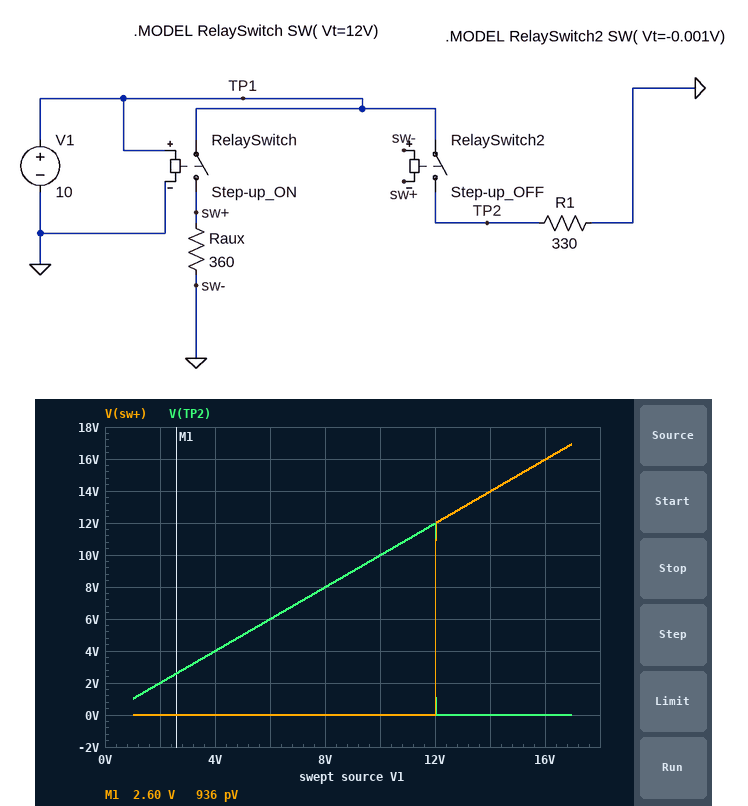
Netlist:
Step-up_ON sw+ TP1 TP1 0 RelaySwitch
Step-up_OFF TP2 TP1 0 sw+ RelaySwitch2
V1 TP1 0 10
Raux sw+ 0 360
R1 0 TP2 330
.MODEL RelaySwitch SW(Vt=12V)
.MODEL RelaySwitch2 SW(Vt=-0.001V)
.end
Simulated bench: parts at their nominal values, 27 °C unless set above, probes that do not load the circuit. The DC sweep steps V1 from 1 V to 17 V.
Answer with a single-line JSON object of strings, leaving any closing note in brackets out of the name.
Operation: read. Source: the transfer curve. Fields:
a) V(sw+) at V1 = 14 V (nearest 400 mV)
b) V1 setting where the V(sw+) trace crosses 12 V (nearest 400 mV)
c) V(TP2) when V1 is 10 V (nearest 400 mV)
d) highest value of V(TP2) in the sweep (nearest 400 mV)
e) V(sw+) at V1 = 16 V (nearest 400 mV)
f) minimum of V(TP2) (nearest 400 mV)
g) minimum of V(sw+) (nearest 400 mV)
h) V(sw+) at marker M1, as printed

{"V(sw+) at V1 = 14 V": "14.0 V", "V1 setting where the V(sw+) trace crosses 12 V": "12.0 V", "V(TP2) when V1 is 10 V": "10.0 V", "highest value of V(TP2) in the sweep": "12.0 V", "V(sw+) at V1 = 16 V": "16.0 V", "minimum of V(TP2)": "0 V", "minimum of V(sw+)": "0 V", "V(sw+) at marker M1, as printed": "936 pV"}
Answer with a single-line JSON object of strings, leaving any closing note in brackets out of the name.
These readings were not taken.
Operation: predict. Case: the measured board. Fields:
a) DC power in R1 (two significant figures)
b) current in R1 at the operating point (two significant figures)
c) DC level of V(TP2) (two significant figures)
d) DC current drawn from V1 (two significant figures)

{"DC power in R1": "300 mW", "current in R1 at the operating point": "30 mA", "DC level of V(TP2)": "10 V", "DC current drawn from V1": "30 mA"}
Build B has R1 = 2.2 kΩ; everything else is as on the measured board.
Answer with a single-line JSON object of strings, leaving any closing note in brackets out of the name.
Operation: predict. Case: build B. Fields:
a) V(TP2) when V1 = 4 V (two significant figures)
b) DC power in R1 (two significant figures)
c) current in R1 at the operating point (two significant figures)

{"V(TP2) when V1 = 4 V": "4.0 V", "DC power in R1": "45 mW", "current in R1 at the operating point": "4.5 mA"}
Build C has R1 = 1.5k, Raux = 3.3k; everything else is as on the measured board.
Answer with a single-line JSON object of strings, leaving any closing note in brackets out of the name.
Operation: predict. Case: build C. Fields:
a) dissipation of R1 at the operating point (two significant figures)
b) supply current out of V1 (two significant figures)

{"dissipation of R1 at the operating point": "67 mW", "supply current out of V1": "6.7 mA"}
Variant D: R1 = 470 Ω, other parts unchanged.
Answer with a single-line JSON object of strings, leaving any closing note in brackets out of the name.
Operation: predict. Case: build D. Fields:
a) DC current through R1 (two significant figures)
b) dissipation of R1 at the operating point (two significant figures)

{"DC current through R1": "21 mA", "dissipation of R1 at the operating point": "210 mW"}
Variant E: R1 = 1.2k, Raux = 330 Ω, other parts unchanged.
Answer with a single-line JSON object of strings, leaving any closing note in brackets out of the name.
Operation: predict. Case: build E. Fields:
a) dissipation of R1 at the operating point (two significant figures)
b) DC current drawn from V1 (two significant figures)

{"dissipation of R1 at the operating point": "83 mW", "DC current drawn from V1": "8.3 mA"}
